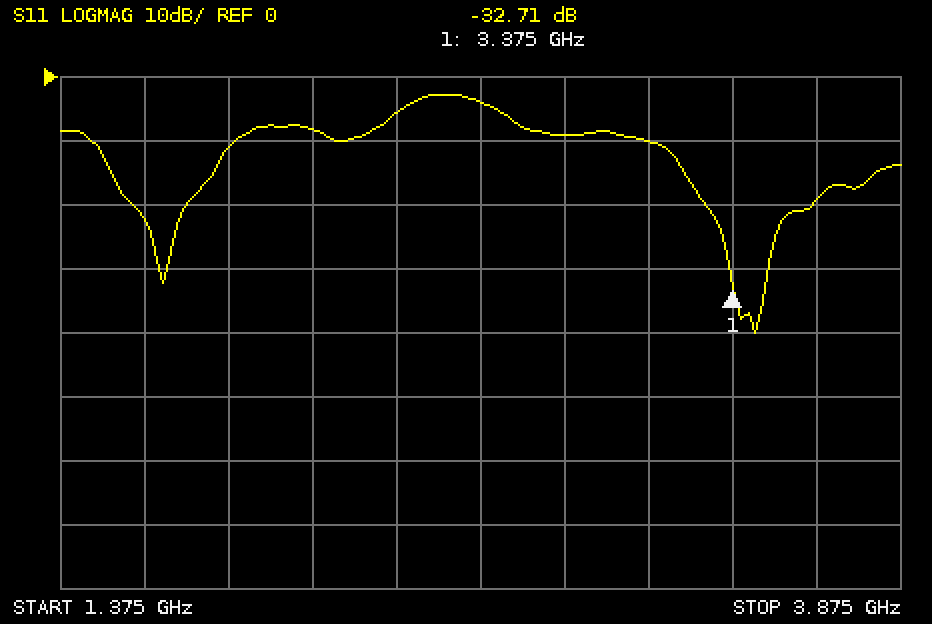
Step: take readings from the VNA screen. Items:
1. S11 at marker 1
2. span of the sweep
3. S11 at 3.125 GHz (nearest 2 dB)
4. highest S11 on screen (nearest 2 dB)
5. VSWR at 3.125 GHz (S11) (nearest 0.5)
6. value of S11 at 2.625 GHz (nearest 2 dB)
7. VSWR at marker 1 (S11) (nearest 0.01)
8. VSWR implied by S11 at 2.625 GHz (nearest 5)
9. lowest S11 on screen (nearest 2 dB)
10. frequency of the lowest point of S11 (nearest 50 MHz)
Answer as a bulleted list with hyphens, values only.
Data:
- -32.71 dB
- 2.5 GHz
- -10 dB
- -2 dB
- 2.0
- -4 dB
- 1.05
- 5
- -40 dB
- 3.45 GHz
